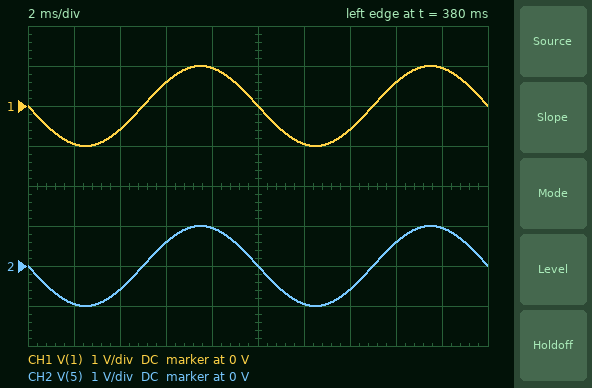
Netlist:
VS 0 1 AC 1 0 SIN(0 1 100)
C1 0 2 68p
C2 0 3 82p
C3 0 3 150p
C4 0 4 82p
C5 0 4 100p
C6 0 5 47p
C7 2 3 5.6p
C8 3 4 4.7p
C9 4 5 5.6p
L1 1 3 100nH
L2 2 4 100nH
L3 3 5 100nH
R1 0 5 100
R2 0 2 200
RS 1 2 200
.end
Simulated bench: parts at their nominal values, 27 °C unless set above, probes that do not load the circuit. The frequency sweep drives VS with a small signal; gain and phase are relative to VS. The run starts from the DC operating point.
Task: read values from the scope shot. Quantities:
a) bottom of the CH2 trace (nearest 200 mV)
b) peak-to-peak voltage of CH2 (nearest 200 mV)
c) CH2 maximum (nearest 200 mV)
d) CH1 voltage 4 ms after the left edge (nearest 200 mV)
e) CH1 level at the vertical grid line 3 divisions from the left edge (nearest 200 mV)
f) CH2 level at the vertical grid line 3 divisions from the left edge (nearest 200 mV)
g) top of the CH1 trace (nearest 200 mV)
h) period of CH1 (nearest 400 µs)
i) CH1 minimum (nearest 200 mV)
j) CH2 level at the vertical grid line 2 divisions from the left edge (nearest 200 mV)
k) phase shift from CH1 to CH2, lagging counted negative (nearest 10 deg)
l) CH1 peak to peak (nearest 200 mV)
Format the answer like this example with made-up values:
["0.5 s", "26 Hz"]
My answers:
["-1.0 V", "2.0 V", "1.0 V", "-600 mV", "600 mV", "600 mV", "1.0 V", "10.0 ms", "-1.0 V", "-600 mV", "0 deg", "2.0 V"]
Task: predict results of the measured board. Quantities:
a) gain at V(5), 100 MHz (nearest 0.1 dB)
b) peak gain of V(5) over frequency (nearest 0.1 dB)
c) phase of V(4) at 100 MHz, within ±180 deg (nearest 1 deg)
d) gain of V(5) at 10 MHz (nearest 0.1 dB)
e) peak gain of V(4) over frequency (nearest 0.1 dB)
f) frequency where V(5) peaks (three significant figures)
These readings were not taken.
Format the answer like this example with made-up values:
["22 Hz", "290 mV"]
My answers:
["-18.8 dB", "13.2 dB", "-75 deg", "1.2 dB", "-6.0 dB", "29.0 MHz"]
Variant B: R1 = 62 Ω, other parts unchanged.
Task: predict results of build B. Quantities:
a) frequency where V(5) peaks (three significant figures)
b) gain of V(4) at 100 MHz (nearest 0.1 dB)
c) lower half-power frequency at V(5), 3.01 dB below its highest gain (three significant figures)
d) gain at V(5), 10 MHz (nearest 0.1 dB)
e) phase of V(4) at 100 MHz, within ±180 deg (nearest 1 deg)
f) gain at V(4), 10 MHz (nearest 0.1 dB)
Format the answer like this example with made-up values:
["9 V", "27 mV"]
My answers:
["29.3 MHz", "-30.9 dB", "22.5 MHz", "1.0 dB", "-73 deg", "-11.1 dB"]
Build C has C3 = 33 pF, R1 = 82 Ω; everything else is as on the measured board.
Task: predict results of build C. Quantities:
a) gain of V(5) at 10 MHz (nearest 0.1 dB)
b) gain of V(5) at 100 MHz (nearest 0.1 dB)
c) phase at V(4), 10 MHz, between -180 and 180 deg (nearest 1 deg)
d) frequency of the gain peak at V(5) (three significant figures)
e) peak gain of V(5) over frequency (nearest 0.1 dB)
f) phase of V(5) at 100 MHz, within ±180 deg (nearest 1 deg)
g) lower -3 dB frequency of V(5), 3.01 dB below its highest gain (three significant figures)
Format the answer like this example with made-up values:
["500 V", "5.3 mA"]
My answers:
["0.7 dB", "-10.0 dB", "131 deg", "35.8 MHz", "8.5 dB", "-131 deg", "26.6 MHz"]
